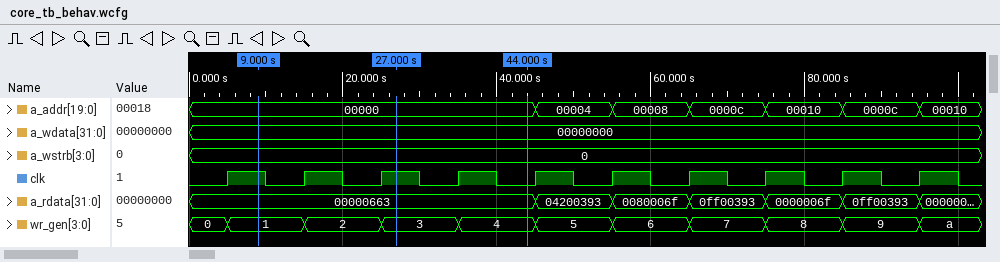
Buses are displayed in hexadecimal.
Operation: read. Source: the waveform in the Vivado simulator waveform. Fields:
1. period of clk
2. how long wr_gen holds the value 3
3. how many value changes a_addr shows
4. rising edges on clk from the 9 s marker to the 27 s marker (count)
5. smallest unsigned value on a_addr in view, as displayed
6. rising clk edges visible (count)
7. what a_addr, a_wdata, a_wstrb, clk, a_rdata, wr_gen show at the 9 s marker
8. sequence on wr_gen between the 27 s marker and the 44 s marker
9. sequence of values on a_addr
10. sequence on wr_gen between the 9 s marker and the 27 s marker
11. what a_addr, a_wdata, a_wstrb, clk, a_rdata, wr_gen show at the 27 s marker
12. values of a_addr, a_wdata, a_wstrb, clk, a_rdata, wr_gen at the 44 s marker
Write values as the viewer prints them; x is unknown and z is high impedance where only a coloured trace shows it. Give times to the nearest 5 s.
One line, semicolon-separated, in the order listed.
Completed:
10 s; 10 s; 6; 2; 00000; 10; a_addr=00000, a_wdata=00000000, a_wstrb=0, clk=1, a_rdata=00000663, wr_gen=1; 3, 4; 00000, 00004, 00008, 0000c, 00010, 0000c, 00010; 1, 2, 3; a_addr=00000, a_wdata=00000000, a_wstrb=0, clk=1, a_rdata=00000663, wr_gen=3; a_addr=00000, a_wdata=00000000, a_wstrb=0, clk=0, a_rdata=00000663, wr_gen=4
